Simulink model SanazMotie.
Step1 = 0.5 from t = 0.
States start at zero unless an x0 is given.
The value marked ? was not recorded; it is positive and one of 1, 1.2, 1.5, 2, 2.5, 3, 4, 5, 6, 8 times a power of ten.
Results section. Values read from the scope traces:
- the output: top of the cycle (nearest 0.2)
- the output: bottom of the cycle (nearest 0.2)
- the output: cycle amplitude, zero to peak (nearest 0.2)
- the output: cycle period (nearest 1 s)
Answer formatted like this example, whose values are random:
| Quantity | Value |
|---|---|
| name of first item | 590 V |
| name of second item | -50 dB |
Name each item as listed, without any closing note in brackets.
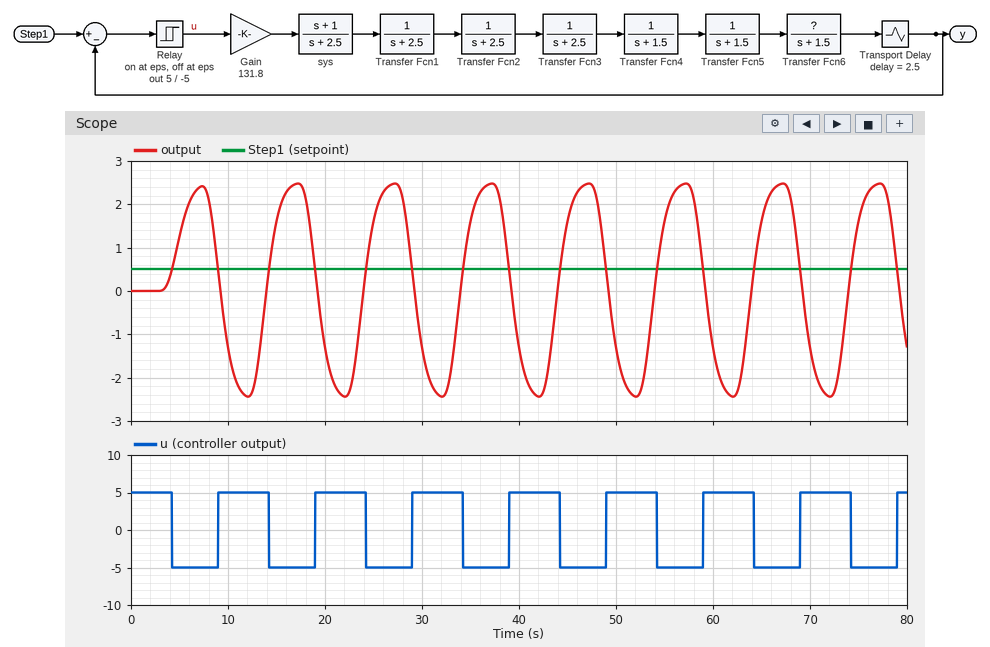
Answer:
| Quantity | Value |
|---|---|
| the output: top of the cycle | 2.4 |
| the output: bottom of the cycle | -2.4 |
| the output: cycle amplitude, zero to peak | 2.4 |
| the output: cycle period | 10 s |
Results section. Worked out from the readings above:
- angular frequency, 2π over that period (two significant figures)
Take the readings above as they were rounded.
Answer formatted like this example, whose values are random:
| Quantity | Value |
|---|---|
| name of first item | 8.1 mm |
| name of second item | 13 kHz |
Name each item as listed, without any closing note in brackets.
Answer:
| Quantity | Value |
|---|---|
| angular frequency, 2π over that period | 0.63 rad/s |
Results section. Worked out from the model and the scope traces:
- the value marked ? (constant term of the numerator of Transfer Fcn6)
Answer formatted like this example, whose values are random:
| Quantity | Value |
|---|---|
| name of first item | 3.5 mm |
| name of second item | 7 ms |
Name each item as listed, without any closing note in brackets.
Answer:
| Quantity | Value |
|---|---|
| the value marked ? | 0.5 |
